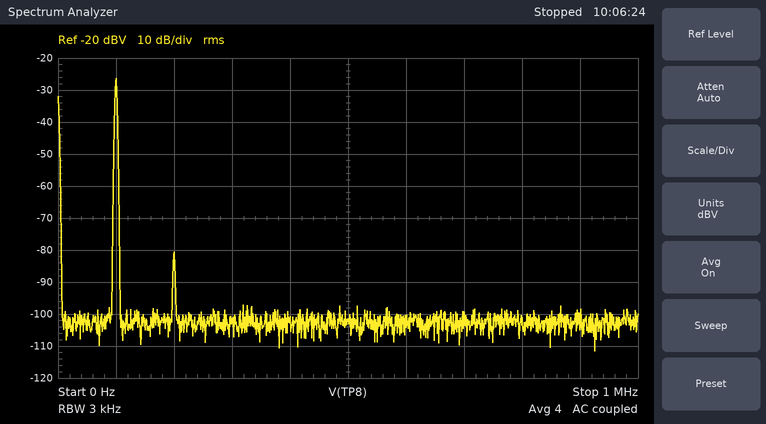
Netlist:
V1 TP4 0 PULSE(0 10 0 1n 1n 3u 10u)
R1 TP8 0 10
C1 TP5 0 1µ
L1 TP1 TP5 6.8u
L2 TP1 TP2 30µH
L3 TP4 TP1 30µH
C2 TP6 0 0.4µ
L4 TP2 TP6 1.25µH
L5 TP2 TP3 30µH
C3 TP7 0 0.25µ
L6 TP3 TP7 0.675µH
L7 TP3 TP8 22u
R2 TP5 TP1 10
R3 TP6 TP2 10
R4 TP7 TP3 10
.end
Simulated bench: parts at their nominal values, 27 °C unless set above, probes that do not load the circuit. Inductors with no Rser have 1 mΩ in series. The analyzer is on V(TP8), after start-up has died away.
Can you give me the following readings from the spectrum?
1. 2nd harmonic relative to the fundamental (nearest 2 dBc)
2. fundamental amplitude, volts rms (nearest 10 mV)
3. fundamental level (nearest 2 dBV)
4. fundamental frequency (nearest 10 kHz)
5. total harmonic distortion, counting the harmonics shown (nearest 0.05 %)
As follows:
-54 dBc
50 mV
-26 dBV
100 kHz
0.20 %
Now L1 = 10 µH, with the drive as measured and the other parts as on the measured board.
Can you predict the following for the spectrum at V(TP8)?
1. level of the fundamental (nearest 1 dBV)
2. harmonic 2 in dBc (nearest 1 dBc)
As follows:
-23 dBV
-56 dBc
